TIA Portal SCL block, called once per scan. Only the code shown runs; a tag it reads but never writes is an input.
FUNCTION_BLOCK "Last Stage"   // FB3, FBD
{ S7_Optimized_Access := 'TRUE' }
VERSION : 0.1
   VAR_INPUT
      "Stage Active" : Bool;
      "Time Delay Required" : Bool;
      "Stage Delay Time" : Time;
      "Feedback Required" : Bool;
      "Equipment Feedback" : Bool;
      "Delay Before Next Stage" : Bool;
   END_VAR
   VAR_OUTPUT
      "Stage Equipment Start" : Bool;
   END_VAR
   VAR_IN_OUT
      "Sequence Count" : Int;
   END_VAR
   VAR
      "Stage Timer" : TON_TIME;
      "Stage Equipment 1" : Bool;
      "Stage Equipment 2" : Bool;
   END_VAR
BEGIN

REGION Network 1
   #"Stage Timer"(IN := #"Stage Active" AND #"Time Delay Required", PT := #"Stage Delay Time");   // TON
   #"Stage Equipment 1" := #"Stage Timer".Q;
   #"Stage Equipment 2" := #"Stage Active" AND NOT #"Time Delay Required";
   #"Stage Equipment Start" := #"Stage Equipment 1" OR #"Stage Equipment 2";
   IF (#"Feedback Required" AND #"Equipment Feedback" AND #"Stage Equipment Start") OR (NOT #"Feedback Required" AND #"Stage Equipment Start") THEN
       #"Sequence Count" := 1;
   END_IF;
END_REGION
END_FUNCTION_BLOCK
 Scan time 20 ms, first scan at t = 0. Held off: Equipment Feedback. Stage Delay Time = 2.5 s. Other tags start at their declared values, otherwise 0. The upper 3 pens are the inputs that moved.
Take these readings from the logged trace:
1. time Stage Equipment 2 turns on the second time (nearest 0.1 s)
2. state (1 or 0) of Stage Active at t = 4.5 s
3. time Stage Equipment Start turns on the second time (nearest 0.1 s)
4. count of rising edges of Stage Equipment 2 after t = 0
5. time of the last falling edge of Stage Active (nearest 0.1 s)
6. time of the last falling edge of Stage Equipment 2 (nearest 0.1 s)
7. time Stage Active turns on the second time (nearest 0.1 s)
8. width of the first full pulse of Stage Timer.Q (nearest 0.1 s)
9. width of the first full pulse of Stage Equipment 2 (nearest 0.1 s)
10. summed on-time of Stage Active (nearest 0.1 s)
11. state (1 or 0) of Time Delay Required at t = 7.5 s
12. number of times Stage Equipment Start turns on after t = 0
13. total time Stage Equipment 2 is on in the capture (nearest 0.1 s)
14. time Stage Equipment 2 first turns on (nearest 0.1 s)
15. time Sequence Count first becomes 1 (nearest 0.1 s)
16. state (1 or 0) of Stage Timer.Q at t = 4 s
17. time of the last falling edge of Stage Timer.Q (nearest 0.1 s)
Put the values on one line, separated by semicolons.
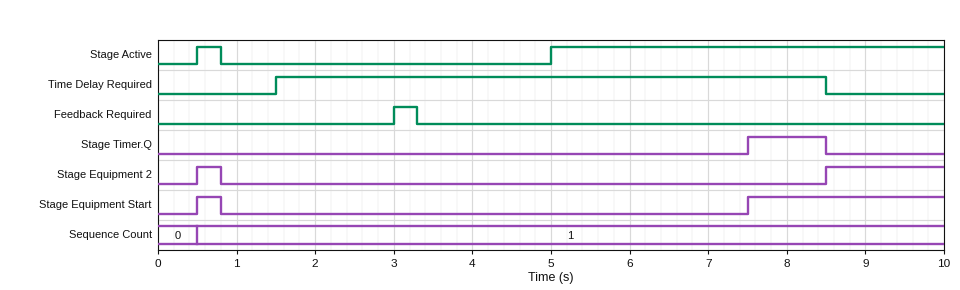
8.5 s; 0; 7.5 s; 2; 0.8 s; 0.8 s; 5.0 s; 1.0 s; 0.3 s; 5.3 s; 1; 2; 1.8 s; 0.5 s; 0.5 s; 0; 8.5 s
